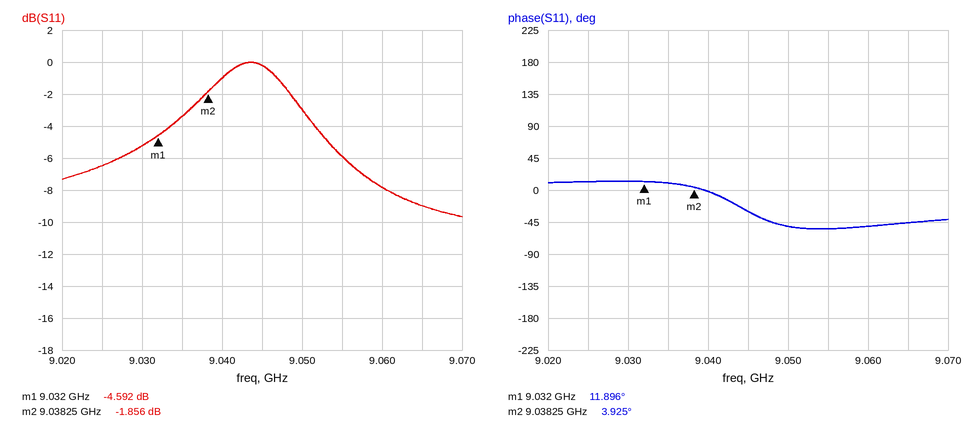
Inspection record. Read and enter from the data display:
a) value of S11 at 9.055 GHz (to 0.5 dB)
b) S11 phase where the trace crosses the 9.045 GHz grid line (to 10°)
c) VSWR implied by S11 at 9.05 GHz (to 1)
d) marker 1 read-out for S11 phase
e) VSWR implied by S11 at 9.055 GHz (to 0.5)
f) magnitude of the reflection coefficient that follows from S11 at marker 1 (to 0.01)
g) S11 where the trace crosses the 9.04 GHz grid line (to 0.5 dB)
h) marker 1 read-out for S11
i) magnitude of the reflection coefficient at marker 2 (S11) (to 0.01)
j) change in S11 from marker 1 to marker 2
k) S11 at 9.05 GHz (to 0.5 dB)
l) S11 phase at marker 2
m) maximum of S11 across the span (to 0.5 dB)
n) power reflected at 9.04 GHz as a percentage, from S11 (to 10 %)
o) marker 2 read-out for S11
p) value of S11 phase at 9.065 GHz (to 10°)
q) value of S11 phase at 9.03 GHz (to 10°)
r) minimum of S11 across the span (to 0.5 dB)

-6.0 dB
-30°
6
11.896°
3.0
0.59
-1.0 dB
-4.592 dB
0.81
2.736 dB
-3.0 dB
3.925°
0.0 dB
80 %
-1.856 dB
-50°
10°
-9.5 dB
